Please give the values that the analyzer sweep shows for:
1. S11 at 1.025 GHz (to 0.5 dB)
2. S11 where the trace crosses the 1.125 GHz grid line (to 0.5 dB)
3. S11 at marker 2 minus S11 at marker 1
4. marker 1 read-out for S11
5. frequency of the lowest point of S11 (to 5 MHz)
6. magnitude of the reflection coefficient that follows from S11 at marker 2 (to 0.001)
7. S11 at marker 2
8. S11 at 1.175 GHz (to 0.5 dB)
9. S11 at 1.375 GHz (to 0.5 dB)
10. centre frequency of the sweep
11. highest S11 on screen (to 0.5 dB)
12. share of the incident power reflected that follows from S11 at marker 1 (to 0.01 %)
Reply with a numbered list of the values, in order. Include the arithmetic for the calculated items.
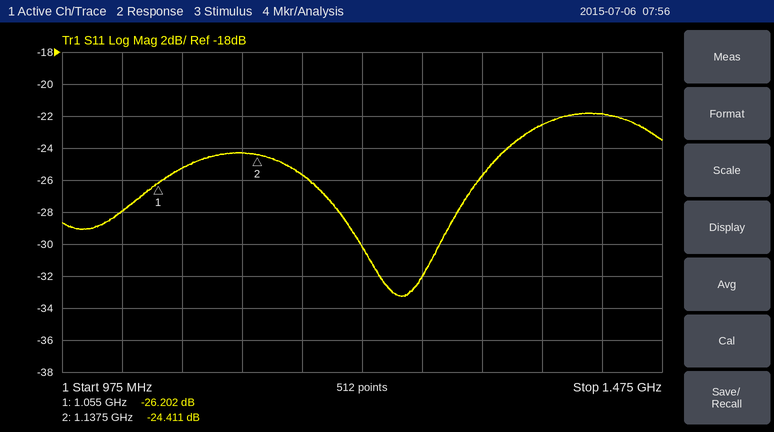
1. -28.0 dB
2. -24.5 dB
3. -24.411 − (-26.202) = 1.791 dB
4. -26.202 dB
5. 1.260 GHz
6. 10^(-24.411/20) ≈ 0.060
7. -24.411 dB
8. -25.5 dB
9. -22.5 dB
10. 1.225 GHz
11. -22.0 dB
12. 10^(-26.202/10) ≈ 0.24 %
